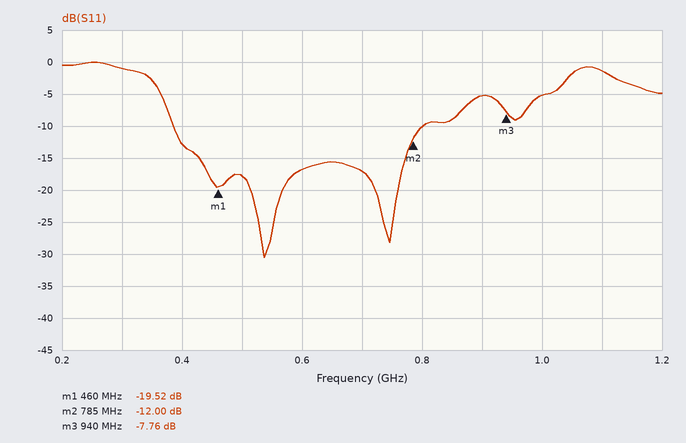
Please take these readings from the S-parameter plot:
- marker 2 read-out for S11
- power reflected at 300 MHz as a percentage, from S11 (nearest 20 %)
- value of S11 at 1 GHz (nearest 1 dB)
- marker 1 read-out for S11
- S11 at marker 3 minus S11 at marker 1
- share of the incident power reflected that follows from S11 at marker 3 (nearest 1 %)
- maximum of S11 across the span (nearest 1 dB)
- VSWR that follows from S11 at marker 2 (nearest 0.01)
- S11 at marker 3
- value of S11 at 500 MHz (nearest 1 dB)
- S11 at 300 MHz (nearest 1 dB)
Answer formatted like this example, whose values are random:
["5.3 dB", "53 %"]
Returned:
["-12.00 dB", "80 %", "-5 dB", "-19.52 dB", "11.76 dB", "17 %", "0 dB", "1.67", "-7.76 dB", "-18 dB", "-1 dB"]
